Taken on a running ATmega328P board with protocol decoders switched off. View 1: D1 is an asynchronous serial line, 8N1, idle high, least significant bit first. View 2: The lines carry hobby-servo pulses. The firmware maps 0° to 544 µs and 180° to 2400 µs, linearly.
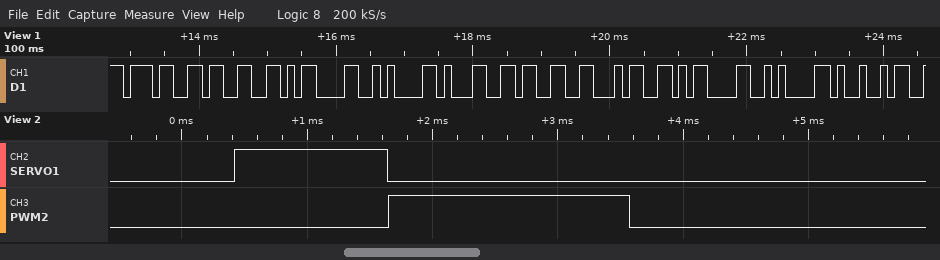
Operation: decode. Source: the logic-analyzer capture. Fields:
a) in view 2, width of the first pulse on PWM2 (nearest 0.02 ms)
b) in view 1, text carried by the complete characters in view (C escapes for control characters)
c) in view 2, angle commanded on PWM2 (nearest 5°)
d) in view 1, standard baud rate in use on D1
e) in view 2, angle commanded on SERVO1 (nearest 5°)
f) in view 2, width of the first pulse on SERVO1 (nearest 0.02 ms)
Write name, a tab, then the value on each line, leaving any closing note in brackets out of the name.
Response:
in view 2, width of the first pulse on PWM2	1.92 ms
in view 1, text carried by the complete characters in view	"73\r\n134\r\nI"
in view 2, angle commanded on PWM2	135°
in view 1, standard baud rate in use on D1	9600 baud
in view 2, angle commanded on SERVO1	65°
in view 2, width of the first pulse on SERVO1	1.22 ms
